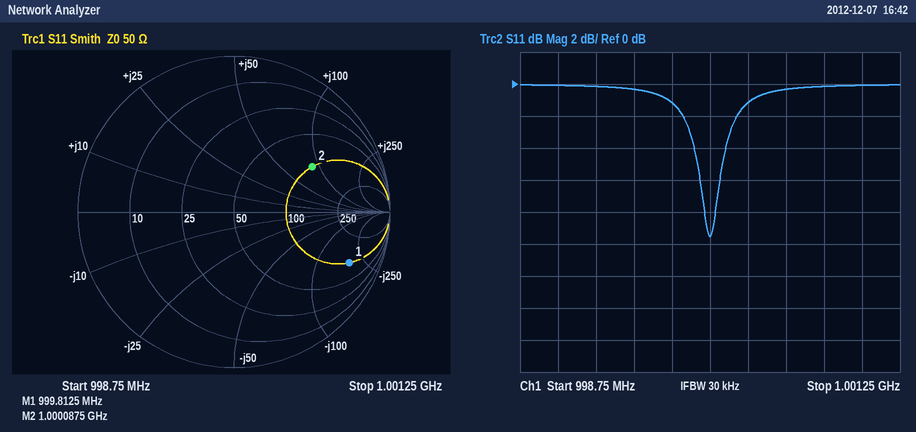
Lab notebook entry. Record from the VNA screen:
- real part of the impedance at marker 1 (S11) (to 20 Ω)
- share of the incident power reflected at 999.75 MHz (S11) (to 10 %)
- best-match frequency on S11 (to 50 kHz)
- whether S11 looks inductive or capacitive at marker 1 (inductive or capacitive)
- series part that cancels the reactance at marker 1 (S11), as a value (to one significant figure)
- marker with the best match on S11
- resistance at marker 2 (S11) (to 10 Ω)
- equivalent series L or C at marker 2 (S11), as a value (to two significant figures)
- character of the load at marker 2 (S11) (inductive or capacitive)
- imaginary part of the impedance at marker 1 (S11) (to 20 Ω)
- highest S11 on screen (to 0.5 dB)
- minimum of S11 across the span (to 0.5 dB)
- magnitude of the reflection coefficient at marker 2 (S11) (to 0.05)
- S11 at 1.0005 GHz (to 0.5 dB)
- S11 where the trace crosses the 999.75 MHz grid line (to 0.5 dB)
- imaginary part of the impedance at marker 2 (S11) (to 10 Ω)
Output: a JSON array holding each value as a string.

["100 Ω", "80 %", "1.00000 GHz", "capacitive", "30 nH", "marker 2", "100 Ω", "14 nH", "inductive", "-180 Ω", "0.0 dB", "-9.5 dB", "0.60", "-0.5 dB", "-1.0 dB", "+90 Ω"]
